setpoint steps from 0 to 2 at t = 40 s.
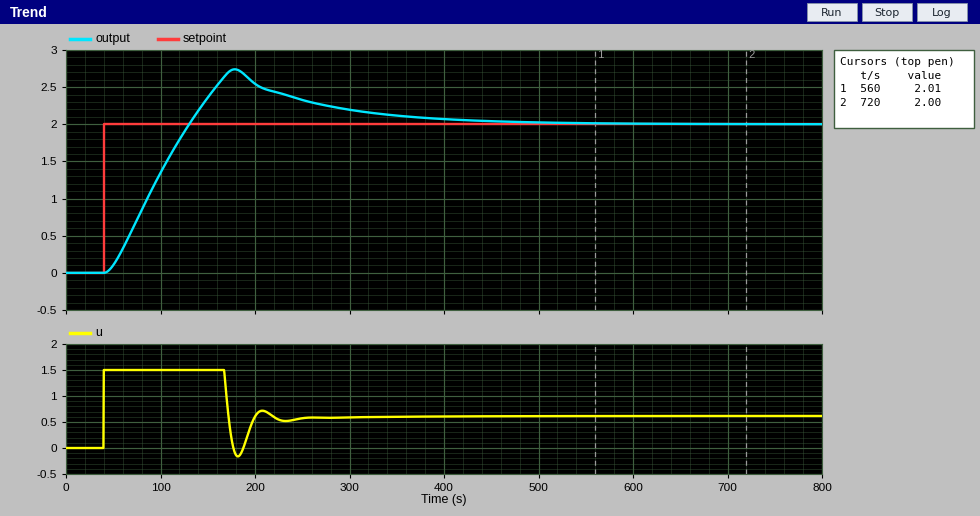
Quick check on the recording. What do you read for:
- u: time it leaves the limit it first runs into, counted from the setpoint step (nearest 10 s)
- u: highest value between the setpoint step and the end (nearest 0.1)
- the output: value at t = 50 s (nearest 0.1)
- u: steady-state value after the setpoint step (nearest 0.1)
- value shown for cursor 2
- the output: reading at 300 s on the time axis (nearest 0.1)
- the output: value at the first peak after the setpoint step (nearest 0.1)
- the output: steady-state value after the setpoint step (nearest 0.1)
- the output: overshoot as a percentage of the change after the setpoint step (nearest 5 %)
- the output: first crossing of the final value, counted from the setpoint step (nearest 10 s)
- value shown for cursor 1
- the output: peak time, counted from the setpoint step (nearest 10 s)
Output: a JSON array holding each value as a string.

["130 s", "1.5", "0.1", "0.6", "2.00", "2.2", "2.7", "2.0", "35 %", "90 s", "2.01", "140 s"]
